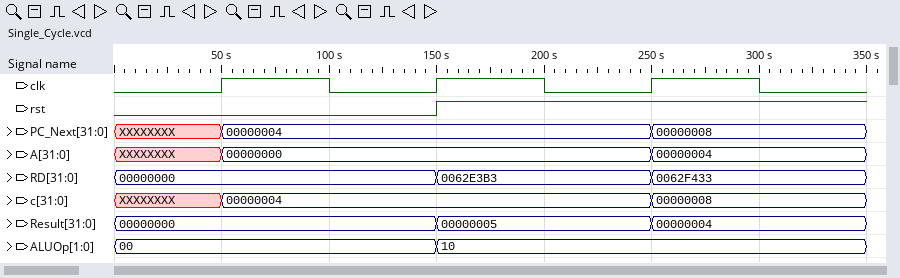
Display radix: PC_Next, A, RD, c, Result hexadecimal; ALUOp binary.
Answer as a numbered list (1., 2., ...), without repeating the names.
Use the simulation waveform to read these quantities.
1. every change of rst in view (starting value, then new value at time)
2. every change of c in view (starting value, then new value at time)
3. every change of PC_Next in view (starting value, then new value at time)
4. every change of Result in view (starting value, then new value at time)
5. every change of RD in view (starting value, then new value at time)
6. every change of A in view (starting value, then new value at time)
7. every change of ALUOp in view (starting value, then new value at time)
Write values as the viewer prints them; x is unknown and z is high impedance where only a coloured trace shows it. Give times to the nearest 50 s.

1. 0, 1 at 150 s
2. XXXXXXXX, 00000004 at 50 s, 00000008 at 250 s
3. XXXXXXXX, 00000004 at 50 s, 00000008 at 250 s
4. 00000000, 00000005 at 150 s, 00000004 at 250 s
5. 00000000, 0062E3B3 at 150 s, 0062F433 at 250 s
6. XXXXXXXX, 00000000 at 50 s, 00000004 at 250 s
7. 00, 10 at 150 s
